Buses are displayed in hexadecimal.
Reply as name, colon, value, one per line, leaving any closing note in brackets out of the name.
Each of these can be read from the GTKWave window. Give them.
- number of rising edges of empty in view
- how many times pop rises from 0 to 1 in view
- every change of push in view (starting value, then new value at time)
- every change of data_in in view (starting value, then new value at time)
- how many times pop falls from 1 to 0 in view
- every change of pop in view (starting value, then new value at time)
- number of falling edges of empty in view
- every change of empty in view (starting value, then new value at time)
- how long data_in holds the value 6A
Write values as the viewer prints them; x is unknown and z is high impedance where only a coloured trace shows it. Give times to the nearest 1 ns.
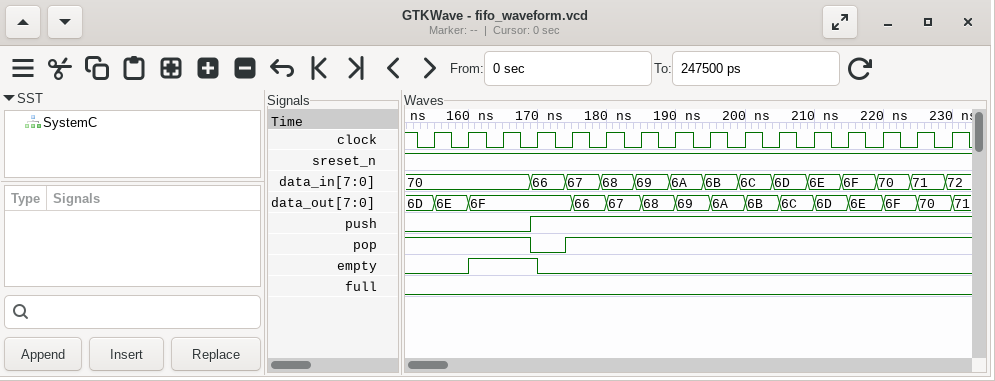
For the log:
number of rising edges of empty in view: 1
how many times pop rises from 0 to 1 in view: 1
every change of push in view: 0, 1 at 169 ns
every change of data_in in view: 70, 66 at 169 ns, 67 at 174 ns, 68 at 179 ns, 69 at 184 ns, 6A at 189 ns, 6B at 194 ns, 6C at 199 ns, 6D at 204 ns, 6E at 209 ns, 6F at 214 ns, 70 at 219 ns, 71 at 224 ns, 72 at 229 ns
how many times pop falls from 1 to 0 in view: 1
every change of pop in view: 1, 0 at 169 ns, 1 at 174 ns
number of falling edges of empty in view: 1
every change of empty in view: 0, 1 at 160 ns, 0 at 170 ns
how long data_in holds the value 6A: 5 ns
